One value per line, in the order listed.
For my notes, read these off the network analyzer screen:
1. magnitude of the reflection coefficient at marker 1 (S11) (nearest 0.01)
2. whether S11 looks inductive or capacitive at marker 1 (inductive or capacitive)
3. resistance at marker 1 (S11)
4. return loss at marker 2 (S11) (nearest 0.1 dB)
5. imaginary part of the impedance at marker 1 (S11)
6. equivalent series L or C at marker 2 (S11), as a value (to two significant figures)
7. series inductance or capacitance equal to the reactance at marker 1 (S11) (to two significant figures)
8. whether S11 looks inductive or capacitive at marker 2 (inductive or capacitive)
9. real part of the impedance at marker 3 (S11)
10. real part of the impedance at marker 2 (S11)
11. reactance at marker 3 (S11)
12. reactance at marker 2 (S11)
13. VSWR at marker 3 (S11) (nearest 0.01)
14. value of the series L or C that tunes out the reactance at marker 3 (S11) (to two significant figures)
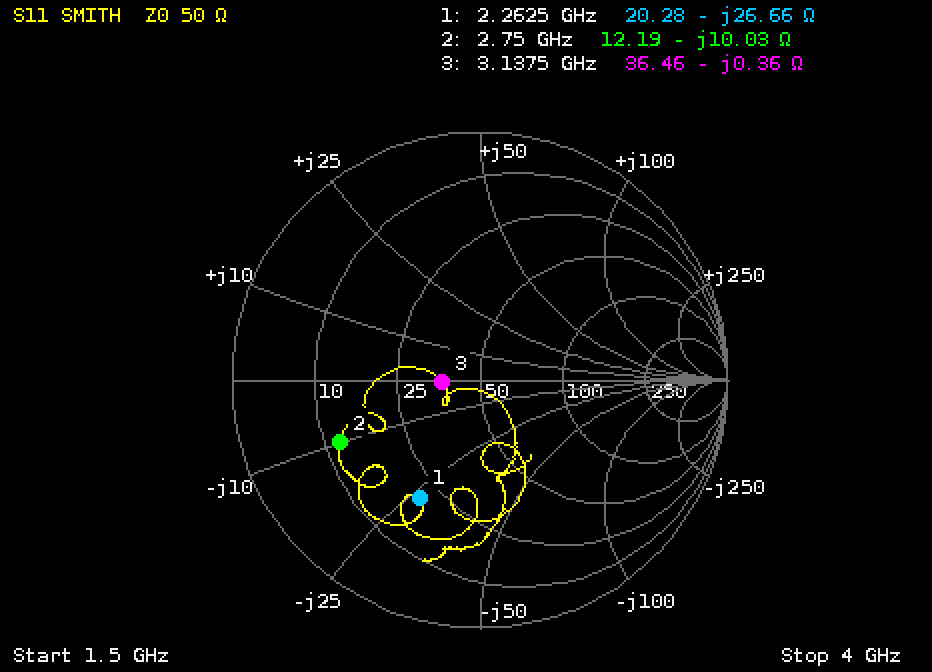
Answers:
0.53
capacitive
20.28 Ω
4.1 dB
-26.66 Ω
5.8 pF
2.6 pF
capacitive
36.46 Ω
12.19 Ω
-0.36 Ω
-10.03 Ω
1.37
18 pH
